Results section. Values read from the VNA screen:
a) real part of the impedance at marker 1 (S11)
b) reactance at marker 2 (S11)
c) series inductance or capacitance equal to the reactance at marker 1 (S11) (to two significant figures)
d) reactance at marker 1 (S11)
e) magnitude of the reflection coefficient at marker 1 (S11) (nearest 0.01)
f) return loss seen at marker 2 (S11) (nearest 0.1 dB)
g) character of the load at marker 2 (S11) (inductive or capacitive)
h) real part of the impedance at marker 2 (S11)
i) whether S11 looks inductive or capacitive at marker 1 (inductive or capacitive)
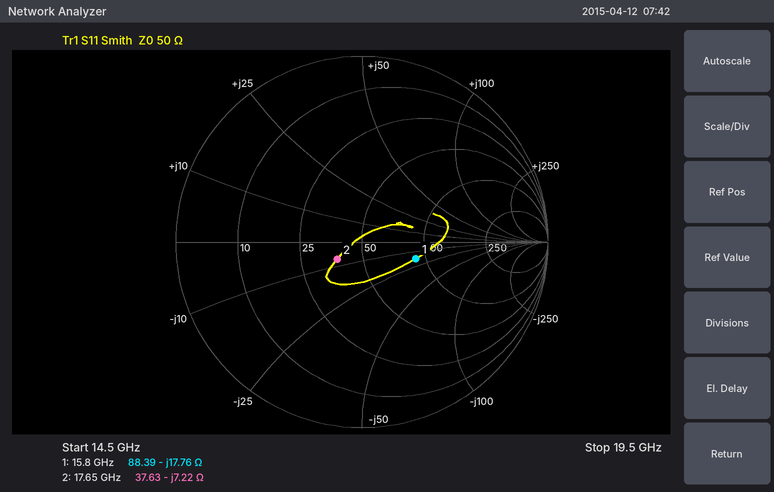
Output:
88.39 Ω
-7.22 Ω
570 fF
-17.76 Ω
0.30
15.8 dB
capacitive
37.63 Ω
capacitive
